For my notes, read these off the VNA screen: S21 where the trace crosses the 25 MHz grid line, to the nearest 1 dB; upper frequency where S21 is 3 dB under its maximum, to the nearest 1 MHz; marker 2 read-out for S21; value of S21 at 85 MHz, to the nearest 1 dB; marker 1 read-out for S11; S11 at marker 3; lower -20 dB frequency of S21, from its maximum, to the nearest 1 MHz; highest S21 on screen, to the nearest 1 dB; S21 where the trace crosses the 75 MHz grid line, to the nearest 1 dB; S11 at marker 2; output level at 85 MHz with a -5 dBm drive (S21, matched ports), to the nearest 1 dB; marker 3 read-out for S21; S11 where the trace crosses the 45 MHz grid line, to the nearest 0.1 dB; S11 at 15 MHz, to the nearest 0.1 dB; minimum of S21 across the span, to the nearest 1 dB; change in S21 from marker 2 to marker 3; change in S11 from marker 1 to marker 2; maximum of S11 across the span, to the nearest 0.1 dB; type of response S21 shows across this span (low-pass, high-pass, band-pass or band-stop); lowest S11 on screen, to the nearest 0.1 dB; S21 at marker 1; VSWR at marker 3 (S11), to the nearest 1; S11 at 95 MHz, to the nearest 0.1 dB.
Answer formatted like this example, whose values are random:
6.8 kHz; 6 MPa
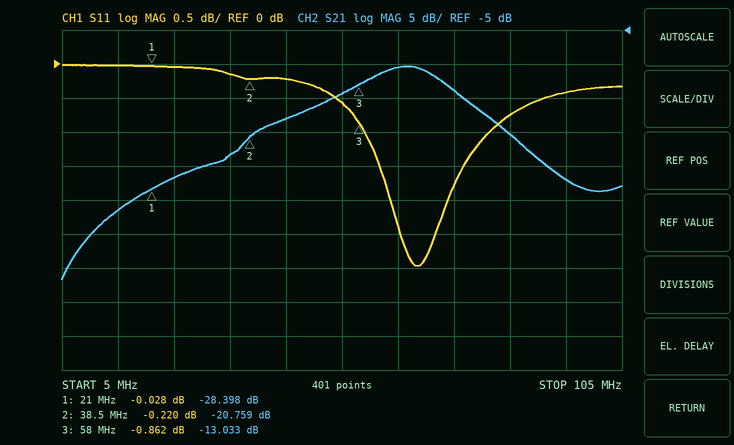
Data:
-27 dB; 74 MHz; -20.759 dB; -20 dB; -0.028 dB; -0.862 dB; 17 MHz; -10 dB; -14 dB; -0.220 dB; -25 dBm; -13.033 dB; -0.2 dB; 0.0 dB; -42 dB; 7.726 dB; -0.192 dB; 0.0 dB; band-pass; -3.0 dB; -28.398 dB; 20; -0.4 dB
